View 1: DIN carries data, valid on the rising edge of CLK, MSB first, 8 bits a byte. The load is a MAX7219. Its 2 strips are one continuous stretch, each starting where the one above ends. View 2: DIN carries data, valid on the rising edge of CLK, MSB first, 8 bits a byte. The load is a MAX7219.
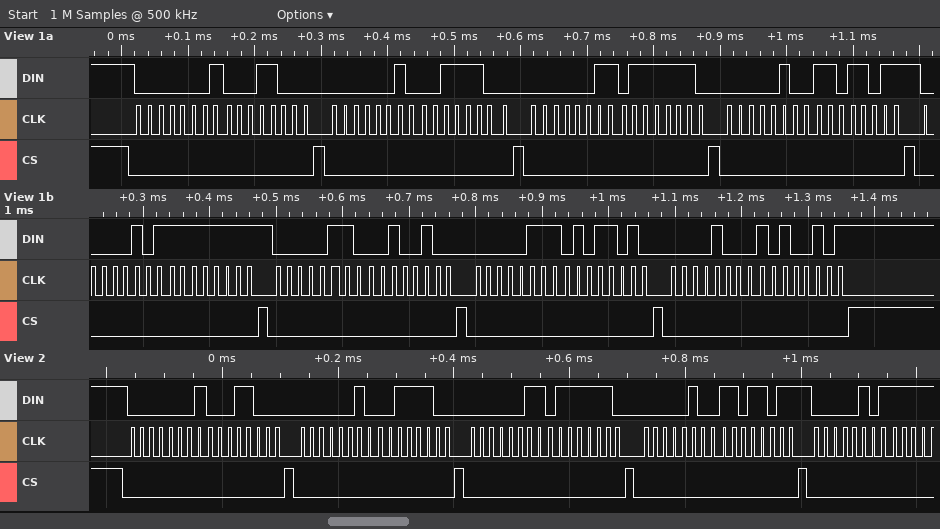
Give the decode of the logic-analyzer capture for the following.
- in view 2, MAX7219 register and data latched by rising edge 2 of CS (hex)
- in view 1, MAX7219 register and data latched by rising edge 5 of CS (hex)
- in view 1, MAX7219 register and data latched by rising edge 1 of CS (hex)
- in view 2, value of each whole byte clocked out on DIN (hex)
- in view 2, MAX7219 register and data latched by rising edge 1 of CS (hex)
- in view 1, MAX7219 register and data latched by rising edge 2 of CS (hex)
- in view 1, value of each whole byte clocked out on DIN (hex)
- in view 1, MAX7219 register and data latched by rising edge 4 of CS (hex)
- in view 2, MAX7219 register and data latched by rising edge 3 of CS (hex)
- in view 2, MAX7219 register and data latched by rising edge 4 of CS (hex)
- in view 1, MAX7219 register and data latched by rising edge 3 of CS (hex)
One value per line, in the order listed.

register 0x2, data 0x3C
register 0x5, data 0xFF
register 0x1, data 0x18
01 18 02 3C 03 7E 04 DB 05
register 0x1, data 0x18
register 0x2, data 0x3C
01 18 02 3C 03 7E 04 DB 05 FF 06 24 07 5A 08 A5
register 0x4, data 0xDB
register 0x3, data 0x7E
register 0x4, data 0xDB
register 0x3, data 0x7E
